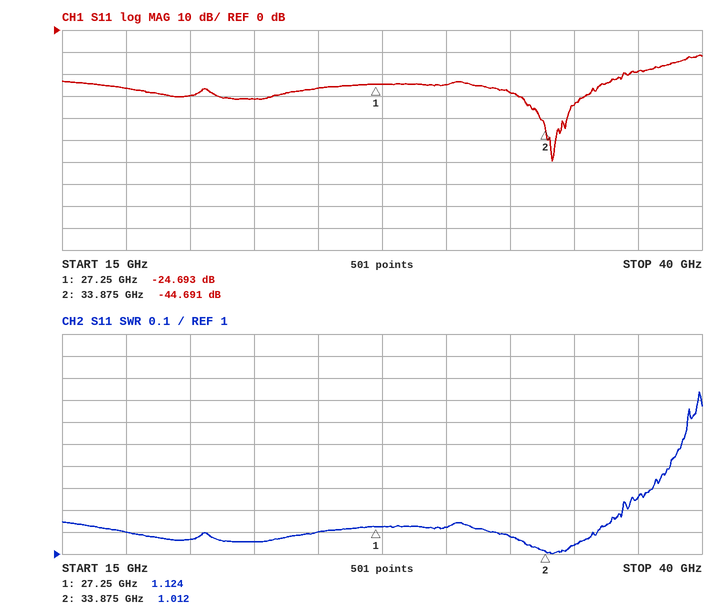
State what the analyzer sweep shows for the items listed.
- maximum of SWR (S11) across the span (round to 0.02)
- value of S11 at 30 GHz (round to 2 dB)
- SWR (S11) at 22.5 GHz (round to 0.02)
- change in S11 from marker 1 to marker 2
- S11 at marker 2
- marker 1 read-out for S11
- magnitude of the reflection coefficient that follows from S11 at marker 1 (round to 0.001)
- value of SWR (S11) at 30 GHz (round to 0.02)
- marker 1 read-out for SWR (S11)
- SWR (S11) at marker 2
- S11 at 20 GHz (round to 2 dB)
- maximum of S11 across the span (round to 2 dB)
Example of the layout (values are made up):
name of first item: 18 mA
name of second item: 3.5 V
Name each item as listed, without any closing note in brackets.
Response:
maximum of SWR (S11) across the span: 1.74
value of S11 at 30 GHz: -24 dB
SWR (S11) at 22.5 GHz: 1.06
change in S11 from marker 1 to marker 2: -19.998 dB
S11 at marker 2: -44.691 dB
marker 1 read-out for S11: -24.693 dB
magnitude of the reflection coefficient that follows from S11 at marker 1: 0.058
value of SWR (S11) at 30 GHz: 1.12
marker 1 read-out for SWR: 1.124
SWR (S11) at marker 2: 1.012
S11 at 20 GHz: -30 dB
maximum of S11 across the span: -12 dB
